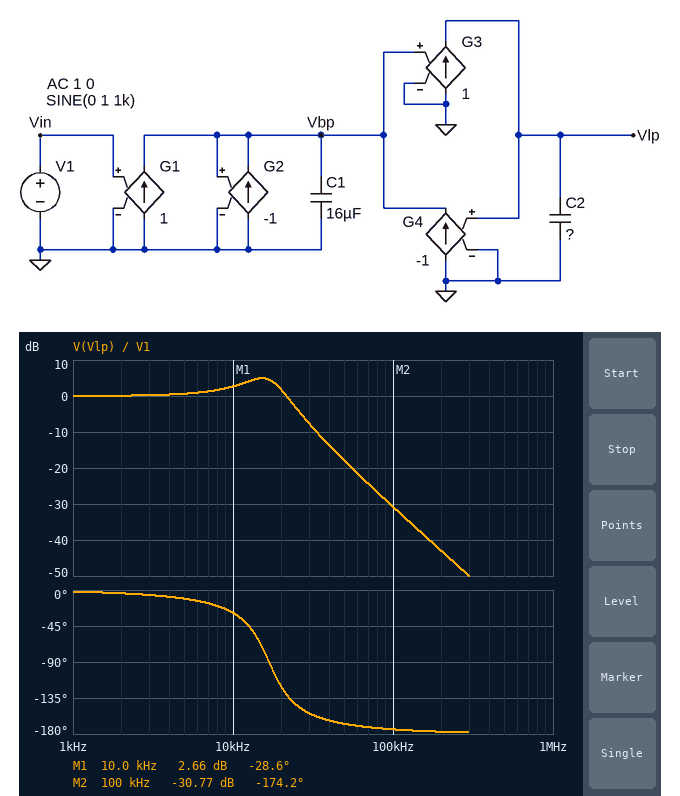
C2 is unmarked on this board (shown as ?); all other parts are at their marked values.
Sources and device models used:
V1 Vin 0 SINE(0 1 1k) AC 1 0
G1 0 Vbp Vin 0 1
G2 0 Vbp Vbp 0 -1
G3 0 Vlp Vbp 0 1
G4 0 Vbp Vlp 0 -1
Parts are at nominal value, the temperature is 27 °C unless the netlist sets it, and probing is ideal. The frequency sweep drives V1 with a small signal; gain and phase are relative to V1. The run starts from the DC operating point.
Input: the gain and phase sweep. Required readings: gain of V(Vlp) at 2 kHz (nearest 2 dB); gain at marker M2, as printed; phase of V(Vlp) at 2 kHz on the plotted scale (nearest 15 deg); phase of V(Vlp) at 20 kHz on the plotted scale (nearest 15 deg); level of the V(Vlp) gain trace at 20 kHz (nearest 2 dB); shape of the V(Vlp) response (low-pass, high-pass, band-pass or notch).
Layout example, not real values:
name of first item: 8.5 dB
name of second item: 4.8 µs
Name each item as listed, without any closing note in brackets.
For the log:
gain of V(Vlp) at 2 kHz: 0 dB
gain at marker M2, as printed: -30.77 dB
phase of V(Vlp) at 2 kHz on the plotted scale: 0 deg
phase of V(Vlp) at 20 kHz on the plotted scale: -120 deg
level of the V(Vlp) gain trace at 20 kHz: 2 dB
shape of the V(Vlp) response: low-pass
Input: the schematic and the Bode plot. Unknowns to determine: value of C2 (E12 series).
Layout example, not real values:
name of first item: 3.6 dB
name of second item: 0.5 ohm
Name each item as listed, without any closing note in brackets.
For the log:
value of C2: 5.6 µF
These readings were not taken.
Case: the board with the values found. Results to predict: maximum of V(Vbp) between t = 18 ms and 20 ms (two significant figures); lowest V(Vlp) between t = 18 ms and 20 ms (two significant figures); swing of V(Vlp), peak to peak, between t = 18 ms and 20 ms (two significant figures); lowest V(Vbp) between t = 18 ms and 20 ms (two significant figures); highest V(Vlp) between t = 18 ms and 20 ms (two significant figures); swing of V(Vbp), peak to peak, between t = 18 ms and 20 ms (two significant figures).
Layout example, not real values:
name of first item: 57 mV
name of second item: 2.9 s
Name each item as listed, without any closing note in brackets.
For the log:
maximum of V(Vbp) between t = 18 ms and 20 ms: 35 mV
lowest V(Vlp) between t = 18 ms and 20 ms: -1.0 V
swing of V(Vlp), peak to peak, between t = 18 ms and 20 ms: 2.0 V
lowest V(Vbp) between t = 18 ms and 20 ms: -35 mV
highest V(Vlp) between t = 18 ms and 20 ms: 1.0 V
swing of V(Vbp), peak to peak, between t = 18 ms and 20 ms: 71 mV
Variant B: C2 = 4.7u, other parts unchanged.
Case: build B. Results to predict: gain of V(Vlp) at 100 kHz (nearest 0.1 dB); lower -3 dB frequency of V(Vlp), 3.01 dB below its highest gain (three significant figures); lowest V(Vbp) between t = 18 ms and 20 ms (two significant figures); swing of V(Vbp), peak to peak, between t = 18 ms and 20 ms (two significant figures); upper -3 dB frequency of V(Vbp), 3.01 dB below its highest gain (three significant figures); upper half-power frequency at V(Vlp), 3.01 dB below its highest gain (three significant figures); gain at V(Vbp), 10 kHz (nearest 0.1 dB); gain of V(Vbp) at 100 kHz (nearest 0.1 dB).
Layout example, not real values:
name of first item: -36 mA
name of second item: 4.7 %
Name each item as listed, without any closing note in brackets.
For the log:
gain of V(Vlp) at 100 kHz: -29.2 dB
lower -3 dB frequency of V(Vlp), 3.01 dB below its highest gain: 10.6 kHz
lowest V(Vbp) between t = 18 ms and 20 ms: -30 mV
swing of V(Vbp), peak to peak, between t = 18 ms and 20 ms: 59 mV
upper -3 dB frequency of V(Vbp), 3.01 dB below its highest gain: 24.0 kHz
upper half-power frequency at V(Vlp), 3.01 dB below its highest gain: 21.5 kHz
gain at V(Vbp), 10 kHz: -8.2 dB
gain of V(Vbp) at 100 kHz: -19.8 dB
